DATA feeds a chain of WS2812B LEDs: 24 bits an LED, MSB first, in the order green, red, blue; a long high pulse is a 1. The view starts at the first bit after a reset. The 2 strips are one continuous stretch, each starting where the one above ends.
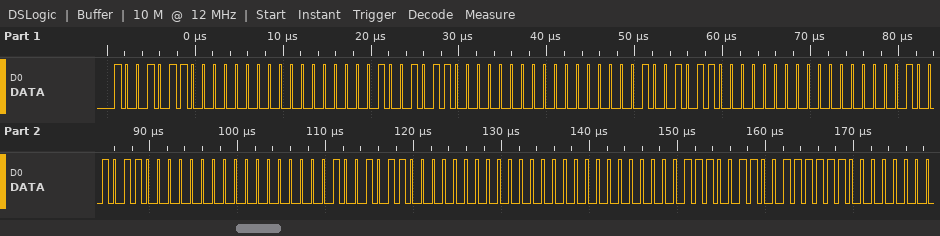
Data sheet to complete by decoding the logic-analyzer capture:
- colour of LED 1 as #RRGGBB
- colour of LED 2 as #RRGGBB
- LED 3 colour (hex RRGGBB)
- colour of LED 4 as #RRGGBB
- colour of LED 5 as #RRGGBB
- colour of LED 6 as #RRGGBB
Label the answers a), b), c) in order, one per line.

a) #009600
b) #009600
c) #009600
d) #009600
e) #009600
f) #E6007E
